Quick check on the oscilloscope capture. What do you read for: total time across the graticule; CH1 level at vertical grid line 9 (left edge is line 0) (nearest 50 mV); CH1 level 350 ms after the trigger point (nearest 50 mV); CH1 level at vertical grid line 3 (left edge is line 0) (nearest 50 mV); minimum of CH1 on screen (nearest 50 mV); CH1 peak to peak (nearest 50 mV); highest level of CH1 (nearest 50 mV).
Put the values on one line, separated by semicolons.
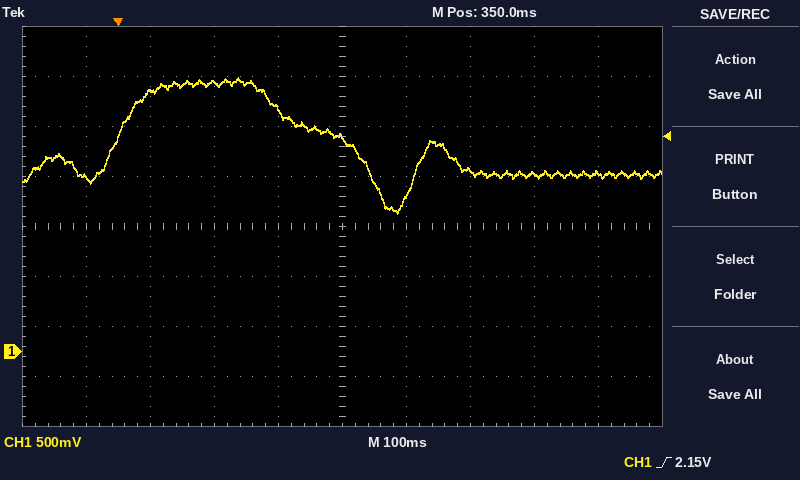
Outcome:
1 s; 1.80 V; 2.15 V; 2.70 V; 1.40 V; 1.35 V; 2.75 V
